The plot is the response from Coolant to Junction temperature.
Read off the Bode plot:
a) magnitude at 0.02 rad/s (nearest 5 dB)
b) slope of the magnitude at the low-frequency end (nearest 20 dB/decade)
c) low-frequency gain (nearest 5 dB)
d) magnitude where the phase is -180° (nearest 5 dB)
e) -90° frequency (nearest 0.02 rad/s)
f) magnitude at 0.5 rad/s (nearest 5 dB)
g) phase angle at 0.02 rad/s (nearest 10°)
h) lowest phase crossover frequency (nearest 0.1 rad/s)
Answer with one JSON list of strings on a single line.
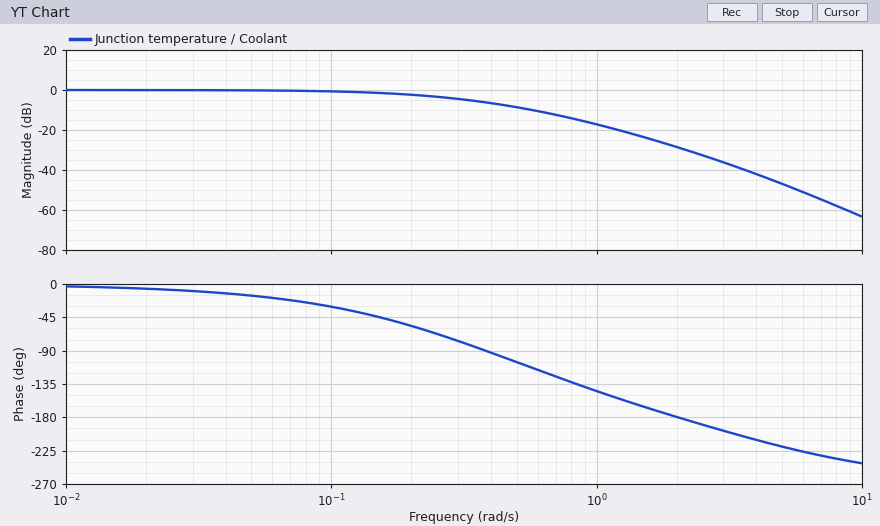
["0 dB", "0 dB/decade", "0 dB", "-30 dB", "0.38 rad/s", "-10 dB", "-10°", "2.0 rad/s"]
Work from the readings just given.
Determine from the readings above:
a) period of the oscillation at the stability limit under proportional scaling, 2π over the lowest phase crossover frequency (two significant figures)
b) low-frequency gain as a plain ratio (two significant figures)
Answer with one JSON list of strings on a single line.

["3.1 s", "1.0"]
